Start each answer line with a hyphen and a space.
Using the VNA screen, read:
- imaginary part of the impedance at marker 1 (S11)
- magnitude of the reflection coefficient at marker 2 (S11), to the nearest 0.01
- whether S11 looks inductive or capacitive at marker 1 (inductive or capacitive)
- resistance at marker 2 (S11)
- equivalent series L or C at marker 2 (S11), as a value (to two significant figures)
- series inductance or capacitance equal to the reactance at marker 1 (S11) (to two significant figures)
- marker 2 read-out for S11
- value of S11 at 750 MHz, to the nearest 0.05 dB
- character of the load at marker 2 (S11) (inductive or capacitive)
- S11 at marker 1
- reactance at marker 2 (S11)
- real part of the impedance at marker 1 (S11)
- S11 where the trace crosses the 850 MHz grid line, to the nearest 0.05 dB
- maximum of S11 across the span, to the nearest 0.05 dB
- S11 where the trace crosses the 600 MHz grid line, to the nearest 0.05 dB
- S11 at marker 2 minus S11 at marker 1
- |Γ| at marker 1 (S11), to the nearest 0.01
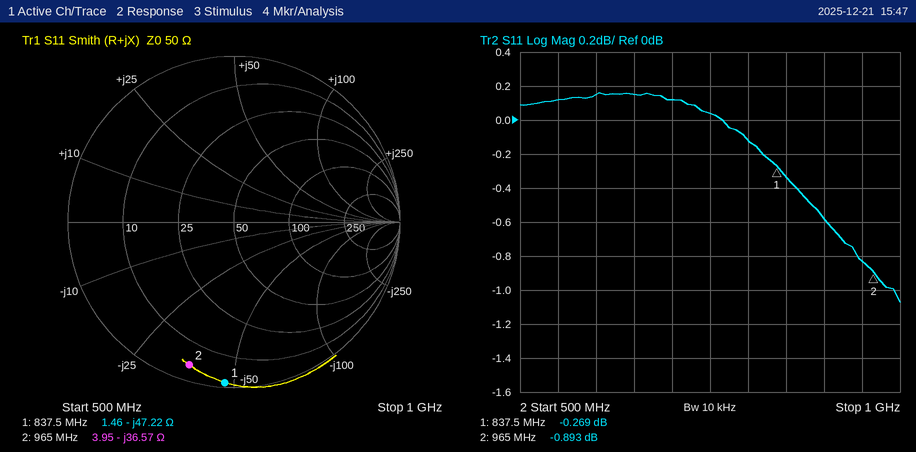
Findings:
- -47.22 Ω
- 0.90
- capacitive
- 3.95 Ω
- 4.5 pF
- 4.0 pF
- -0.893 dB
- 0.05 dB
- capacitive
- -0.269 dB
- -36.57 Ω
- 1.46 Ω
- -0.35 dB
- 0.15 dB
- 0.15 dB
- -0.624 dB
- 0.97
